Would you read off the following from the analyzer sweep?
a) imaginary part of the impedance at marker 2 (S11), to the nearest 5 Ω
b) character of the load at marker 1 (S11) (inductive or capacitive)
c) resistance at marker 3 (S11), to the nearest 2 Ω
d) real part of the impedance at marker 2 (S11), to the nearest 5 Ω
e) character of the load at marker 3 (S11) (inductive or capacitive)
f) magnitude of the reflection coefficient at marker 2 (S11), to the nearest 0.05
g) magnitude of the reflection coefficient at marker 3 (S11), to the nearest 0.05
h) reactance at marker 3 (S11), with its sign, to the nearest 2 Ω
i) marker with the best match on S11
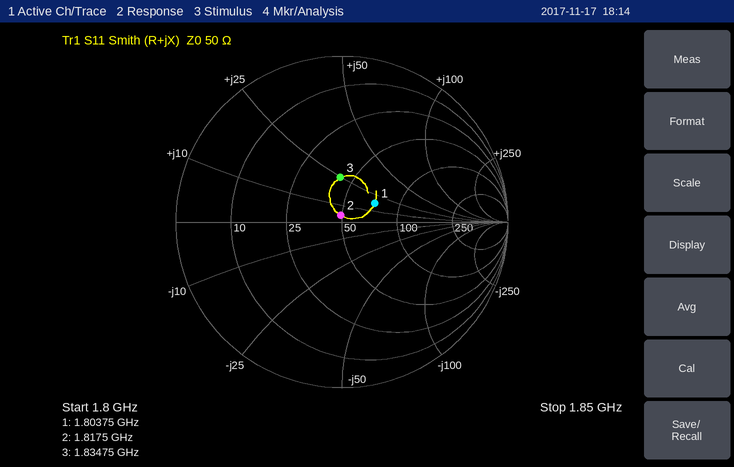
+5 Ω
inductive
42 Ω
50 Ω
inductive
0.05
0.25
+24 Ω
marker 2
